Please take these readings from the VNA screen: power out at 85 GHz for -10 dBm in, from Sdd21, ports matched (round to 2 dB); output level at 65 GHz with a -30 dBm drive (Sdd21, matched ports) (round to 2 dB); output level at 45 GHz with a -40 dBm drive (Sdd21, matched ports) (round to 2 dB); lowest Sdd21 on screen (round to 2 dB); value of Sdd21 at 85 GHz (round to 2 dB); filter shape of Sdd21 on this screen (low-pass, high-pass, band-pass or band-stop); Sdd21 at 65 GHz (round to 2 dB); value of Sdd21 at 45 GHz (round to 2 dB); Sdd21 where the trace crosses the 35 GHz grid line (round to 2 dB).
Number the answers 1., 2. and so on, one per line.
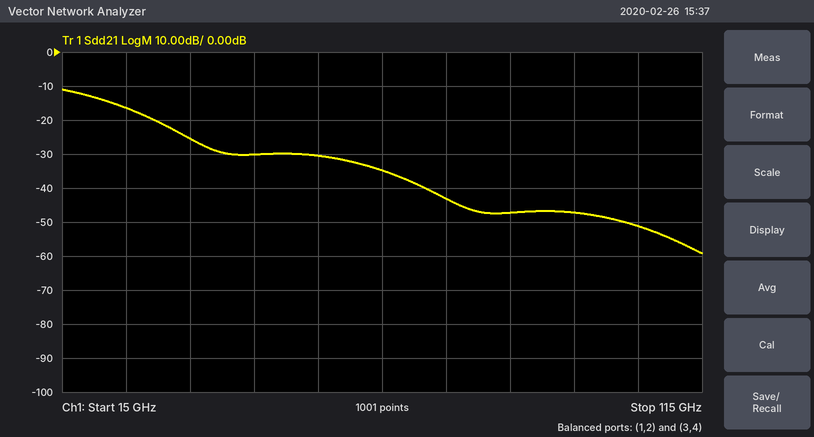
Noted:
1. -58 dBm
2. -64 dBm
3. -70 dBm
4. -60 dB
5. -48 dB
6. low-pass
7. -34 dB
8. -30 dB
9. -26 dB
